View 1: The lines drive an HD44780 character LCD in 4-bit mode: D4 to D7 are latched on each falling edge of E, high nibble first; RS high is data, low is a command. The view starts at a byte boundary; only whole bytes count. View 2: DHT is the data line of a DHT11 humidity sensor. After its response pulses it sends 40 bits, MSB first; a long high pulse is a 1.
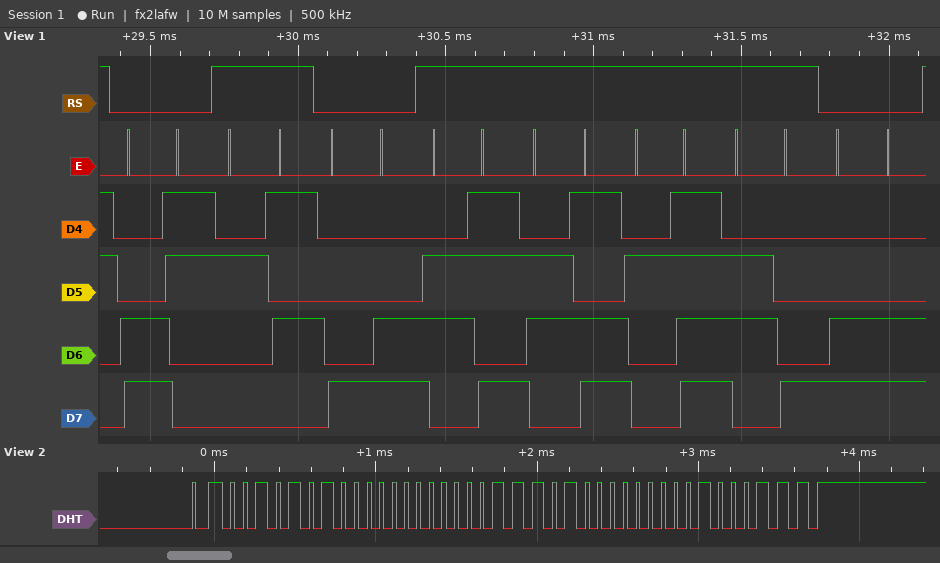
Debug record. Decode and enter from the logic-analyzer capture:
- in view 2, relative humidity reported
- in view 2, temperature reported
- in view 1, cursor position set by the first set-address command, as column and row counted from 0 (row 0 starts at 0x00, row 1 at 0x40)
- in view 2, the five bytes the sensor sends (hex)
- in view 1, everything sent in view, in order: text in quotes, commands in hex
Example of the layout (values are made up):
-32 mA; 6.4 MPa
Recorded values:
42 %; 29.0 °C; column 3, row 1; 2A 00 1D 00 47; 0xC3 "%" 0x8C "km/h" 0xCC
